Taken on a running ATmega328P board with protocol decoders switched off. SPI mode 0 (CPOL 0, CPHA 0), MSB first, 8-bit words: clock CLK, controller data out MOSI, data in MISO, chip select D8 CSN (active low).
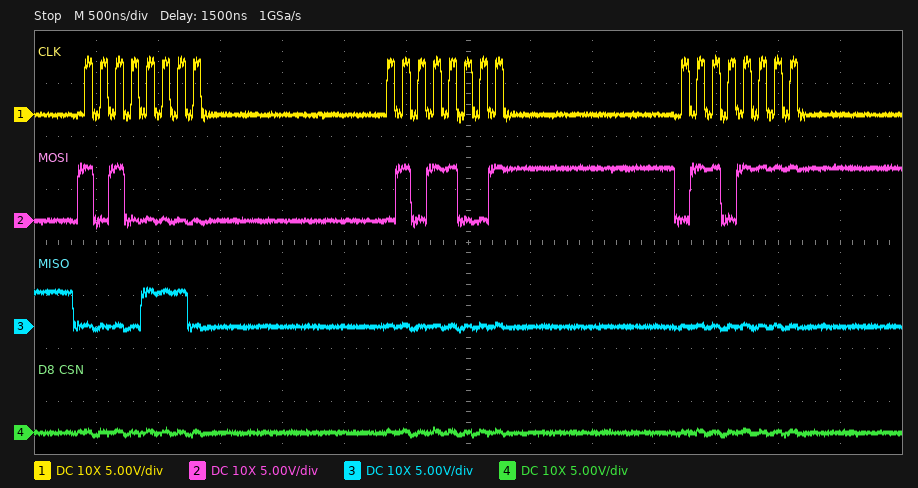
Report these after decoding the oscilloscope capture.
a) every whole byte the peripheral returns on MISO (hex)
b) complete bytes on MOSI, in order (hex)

0E 00 00
A0 59 6F
